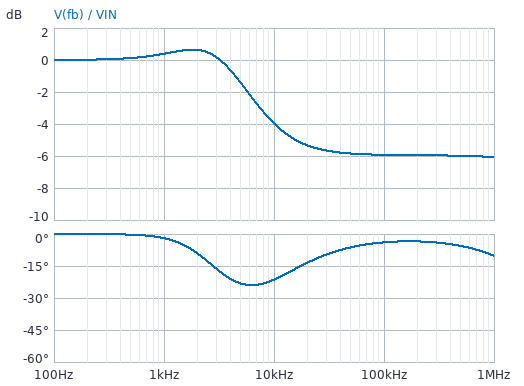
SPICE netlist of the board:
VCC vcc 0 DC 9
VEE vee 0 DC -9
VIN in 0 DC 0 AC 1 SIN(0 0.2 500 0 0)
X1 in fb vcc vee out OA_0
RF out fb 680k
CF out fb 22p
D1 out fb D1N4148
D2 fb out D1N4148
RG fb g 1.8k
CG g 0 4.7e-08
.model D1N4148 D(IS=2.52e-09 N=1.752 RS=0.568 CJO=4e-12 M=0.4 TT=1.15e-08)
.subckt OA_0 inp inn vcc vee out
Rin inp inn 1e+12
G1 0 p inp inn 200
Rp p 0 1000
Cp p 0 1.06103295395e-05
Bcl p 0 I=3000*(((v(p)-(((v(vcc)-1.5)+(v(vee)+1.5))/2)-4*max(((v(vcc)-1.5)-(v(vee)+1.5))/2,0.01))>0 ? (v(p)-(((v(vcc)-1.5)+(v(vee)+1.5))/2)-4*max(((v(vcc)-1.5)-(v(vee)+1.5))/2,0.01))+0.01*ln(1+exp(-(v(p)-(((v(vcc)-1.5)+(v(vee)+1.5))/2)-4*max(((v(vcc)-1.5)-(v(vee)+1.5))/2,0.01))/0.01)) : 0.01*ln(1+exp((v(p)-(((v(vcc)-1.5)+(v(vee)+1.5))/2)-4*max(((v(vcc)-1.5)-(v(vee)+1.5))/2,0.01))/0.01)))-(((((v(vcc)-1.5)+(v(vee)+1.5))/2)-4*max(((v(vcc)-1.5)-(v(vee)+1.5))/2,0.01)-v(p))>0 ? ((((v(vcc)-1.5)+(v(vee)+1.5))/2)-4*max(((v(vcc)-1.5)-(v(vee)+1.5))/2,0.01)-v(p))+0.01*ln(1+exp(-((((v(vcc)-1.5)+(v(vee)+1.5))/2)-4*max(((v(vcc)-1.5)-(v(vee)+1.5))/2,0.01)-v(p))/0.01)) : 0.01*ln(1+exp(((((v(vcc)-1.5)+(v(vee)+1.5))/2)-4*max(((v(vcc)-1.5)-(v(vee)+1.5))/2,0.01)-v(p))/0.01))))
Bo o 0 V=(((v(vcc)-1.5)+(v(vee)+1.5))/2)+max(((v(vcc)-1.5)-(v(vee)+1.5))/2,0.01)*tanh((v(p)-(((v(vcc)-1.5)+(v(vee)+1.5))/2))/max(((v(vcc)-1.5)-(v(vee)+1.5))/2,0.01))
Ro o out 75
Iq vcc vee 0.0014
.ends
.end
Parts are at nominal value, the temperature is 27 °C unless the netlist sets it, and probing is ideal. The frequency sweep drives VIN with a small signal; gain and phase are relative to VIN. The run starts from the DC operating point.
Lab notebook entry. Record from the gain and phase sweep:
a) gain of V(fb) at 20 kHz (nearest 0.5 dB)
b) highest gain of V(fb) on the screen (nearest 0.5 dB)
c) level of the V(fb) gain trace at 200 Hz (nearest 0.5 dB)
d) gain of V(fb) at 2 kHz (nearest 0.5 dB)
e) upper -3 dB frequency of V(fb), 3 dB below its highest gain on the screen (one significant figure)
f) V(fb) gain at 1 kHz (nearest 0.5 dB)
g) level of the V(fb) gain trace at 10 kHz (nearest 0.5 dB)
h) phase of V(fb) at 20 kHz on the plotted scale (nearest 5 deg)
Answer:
-5.5 dB
0.5 dB
0 dB
0.5 dB
6 kHz
0.5 dB
-4.0 dB
-15 deg
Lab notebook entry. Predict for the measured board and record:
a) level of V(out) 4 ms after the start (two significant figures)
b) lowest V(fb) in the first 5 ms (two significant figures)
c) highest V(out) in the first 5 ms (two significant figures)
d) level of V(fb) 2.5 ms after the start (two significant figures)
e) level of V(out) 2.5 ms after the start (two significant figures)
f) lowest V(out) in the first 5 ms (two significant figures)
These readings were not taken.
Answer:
420 mV
-200 mV
580 mV
200 mV
560 mV
-580 mV
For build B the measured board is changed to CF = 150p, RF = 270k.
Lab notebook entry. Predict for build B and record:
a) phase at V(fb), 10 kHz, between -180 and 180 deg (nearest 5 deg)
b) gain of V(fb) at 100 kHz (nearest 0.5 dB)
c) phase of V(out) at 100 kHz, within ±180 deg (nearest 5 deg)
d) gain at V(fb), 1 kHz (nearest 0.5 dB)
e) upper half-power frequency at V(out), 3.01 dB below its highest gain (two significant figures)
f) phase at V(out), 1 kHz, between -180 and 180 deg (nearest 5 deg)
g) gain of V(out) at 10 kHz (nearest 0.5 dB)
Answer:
-5 deg
-1.5 dB
-80 deg
0 dB
5.9 kHz
45 deg
33.0 dB
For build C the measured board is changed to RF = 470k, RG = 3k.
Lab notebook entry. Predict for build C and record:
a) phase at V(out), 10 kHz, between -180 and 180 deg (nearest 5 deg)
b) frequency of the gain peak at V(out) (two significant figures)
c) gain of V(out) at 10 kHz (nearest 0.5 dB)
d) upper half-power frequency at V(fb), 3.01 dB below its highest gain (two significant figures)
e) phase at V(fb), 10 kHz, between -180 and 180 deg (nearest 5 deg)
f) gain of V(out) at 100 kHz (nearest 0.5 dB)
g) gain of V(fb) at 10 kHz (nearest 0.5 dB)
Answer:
-50 deg
2.9 kHz
39.0 dB
15 kHz
-15 deg
21.0 dB
-2.0 dB
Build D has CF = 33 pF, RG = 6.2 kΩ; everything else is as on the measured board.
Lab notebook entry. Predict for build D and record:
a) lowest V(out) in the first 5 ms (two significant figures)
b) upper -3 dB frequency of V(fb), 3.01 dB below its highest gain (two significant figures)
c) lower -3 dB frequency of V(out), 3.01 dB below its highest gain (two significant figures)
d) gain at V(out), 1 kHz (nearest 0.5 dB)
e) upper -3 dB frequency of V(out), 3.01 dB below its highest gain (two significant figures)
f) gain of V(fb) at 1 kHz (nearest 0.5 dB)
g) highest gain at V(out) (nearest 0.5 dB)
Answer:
-600 mV
2.1 MHz
460 Hz
39.0 dB
6.0 kHz
0 dB
39.5 dB
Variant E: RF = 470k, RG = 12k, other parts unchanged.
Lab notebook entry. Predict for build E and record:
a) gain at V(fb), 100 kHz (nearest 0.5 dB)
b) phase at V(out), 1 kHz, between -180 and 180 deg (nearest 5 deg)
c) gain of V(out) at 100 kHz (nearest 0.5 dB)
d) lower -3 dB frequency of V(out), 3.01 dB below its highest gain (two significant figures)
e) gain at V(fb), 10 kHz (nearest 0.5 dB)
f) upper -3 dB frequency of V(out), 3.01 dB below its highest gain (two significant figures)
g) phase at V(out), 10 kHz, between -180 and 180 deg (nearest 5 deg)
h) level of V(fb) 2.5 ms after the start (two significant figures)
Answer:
-1.0 dB
10 deg
12.0 dB
270 Hz
-0.5 dB
11 kHz
-40 deg
200 mV
